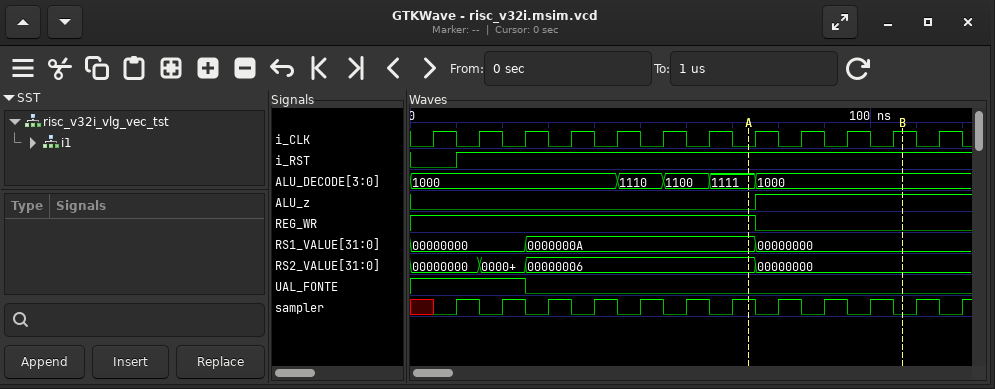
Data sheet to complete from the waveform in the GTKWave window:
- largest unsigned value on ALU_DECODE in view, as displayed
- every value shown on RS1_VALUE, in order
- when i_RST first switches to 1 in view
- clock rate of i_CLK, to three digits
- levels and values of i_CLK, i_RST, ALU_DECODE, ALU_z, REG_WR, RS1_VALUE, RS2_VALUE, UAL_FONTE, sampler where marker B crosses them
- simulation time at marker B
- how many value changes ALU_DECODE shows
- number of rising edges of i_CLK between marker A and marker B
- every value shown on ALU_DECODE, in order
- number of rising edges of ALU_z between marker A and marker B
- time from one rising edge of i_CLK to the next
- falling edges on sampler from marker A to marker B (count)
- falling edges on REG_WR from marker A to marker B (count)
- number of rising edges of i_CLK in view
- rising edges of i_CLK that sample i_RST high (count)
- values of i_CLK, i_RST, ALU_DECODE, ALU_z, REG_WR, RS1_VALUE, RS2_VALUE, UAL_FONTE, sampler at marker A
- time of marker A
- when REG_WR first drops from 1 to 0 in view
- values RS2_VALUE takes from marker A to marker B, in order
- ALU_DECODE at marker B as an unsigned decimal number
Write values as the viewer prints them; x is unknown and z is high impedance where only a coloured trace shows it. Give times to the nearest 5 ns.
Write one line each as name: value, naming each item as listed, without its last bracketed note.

largest unsigned value on ALU_DECODE in view, as displayed: 1111
every value shown on RS1_VALUE, in order: 00000000, 0000000A, 00000000
when i_RST first switches to 1 in view: 10 ns
clock rate of i_CLK, to three digits: 100 MHz
levels and values of i_CLK, i_RST, ALU_DECODE, ALU_z, REG_WR, RS1_VALUE, RS2_VALUE, UAL_FONTE, sampler where marker B crosses them: i_CLK=1, i_RST=1, ALU_DECODE=1000, ALU_z=1, REG_WR=0, RS1_VALUE=00000000, RS2_VALUE=00000000, UAL_FONTE=0, sampler=0
simulation time at marker B: 105 ns
how many value changes ALU_DECODE shows: 4
number of rising edges of i_CLK between marker A and marker B: 4
every value shown on ALU_DECODE, in order: 1000, 1110, 1100, 1111, 1000
number of rising edges of ALU_z between marker A and marker B: 1
time from one rising edge of i_CLK to the next: 10 ns
falling edges on sampler from marker A to marker B: 4
falling edges on REG_WR from marker A to marker B: 1
number of rising edges of i_CLK in view: 12
rising edges of i_CLK that sample i_RST high: 11
values of i_CLK, i_RST, ALU_DECODE, ALU_z, REG_WR, RS1_VALUE, RS2_VALUE, UAL_FONTE, sampler at marker A: i_CLK=0, i_RST=1, ALU_DECODE=1111, ALU_z=0, REG_WR=1, RS1_VALUE=0000000A, RS2_VALUE=00000006, UAL_FONTE=0, sampler=1
time of marker A: 75 ns
when REG_WR first drops from 1 to 0 in view: 75 ns
values RS2_VALUE takes from marker A to marker B, in order: 00000006, 00000000
ALU_DECODE at marker B as an unsigned decimal number: 8
